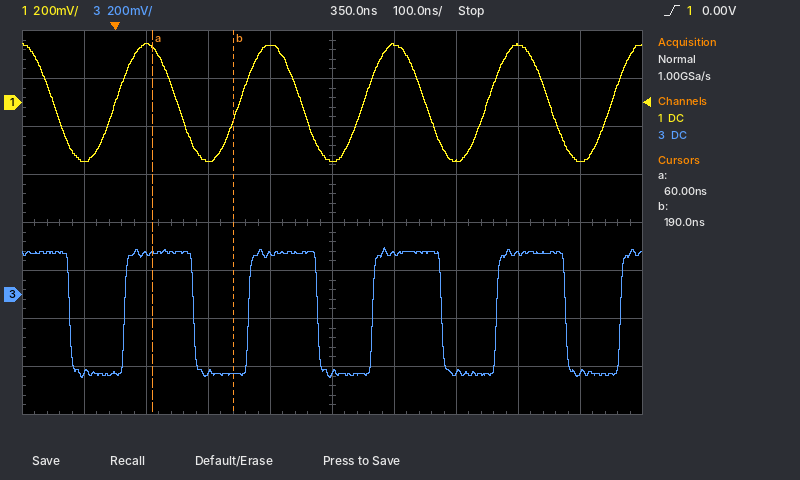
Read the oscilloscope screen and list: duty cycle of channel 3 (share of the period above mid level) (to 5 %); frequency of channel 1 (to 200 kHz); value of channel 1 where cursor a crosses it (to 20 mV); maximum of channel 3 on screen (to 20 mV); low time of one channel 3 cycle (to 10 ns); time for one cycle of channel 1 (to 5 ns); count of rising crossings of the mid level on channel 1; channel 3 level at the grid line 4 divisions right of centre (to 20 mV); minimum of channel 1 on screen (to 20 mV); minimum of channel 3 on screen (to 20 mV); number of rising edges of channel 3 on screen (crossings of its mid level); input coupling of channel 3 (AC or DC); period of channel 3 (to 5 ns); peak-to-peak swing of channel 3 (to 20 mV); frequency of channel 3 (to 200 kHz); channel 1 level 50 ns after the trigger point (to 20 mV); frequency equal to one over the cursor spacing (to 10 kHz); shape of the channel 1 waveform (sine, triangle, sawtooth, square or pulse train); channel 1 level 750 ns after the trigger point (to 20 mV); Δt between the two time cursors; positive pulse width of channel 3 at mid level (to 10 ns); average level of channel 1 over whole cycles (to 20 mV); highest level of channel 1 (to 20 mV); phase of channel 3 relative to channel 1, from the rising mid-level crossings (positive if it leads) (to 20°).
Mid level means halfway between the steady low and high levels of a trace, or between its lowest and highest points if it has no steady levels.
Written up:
55 %
5.0 MHz
220 mV
200 mV
90 ns
200 ns
5
-320 mV
-240 mV
-340 mV
5
DC
200 ns
540 mV
5.0 MHz
240 mV
7.69 MHz
sine
-240 mV
130 ns
110 ns
0 mV
240 mV
-20°
